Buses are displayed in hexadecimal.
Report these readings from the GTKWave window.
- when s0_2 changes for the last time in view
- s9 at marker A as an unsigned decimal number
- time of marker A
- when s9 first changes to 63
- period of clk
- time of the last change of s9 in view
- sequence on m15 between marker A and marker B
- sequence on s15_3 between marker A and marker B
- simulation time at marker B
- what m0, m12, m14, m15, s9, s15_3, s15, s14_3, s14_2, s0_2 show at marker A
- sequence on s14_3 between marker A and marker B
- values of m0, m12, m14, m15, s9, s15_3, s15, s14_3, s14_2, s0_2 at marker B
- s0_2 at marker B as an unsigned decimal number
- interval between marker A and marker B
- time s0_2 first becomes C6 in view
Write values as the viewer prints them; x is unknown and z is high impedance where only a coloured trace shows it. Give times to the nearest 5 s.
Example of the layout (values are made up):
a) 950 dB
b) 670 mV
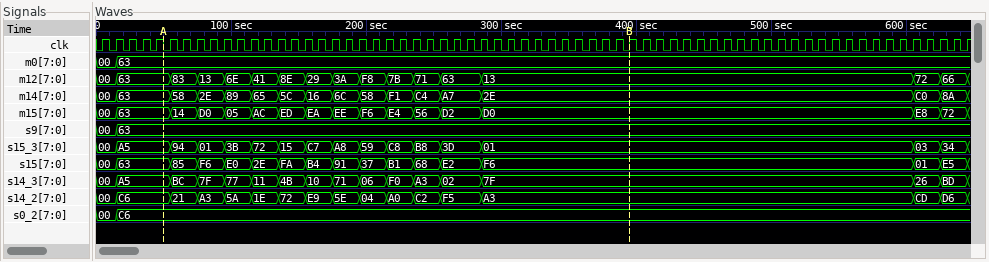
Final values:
a) 15 s
b) 99
c) 50 s
d) 15 s
e) 10 s
f) 15 s
g) 63, 14, D0, 05, AC, ED, EA, EE, F6, E4, 56, D2, D0
h) A5, 94, 01, 3B, 72, 15, C7, A8, 59, C8, B8, 3D, 01
i) 395 s
j) m0=63, m12=63, m14=63, m15=63, s9=63, s15_3=A5, s15=63, s14_3=A5, s14_2=C6, s0_2=C6
k) A5, BC, 7F, 77, 11, 4B, 10, 71, 06, F0, A3, 02, 7F
l) m0=63, m12=13, m14=2E, m15=D0, s9=63, s15_3=01, s15=F6, s14_3=7F, s14_2=A3, s0_2=C6
m) 198
n) 345 s
o) 15 s
